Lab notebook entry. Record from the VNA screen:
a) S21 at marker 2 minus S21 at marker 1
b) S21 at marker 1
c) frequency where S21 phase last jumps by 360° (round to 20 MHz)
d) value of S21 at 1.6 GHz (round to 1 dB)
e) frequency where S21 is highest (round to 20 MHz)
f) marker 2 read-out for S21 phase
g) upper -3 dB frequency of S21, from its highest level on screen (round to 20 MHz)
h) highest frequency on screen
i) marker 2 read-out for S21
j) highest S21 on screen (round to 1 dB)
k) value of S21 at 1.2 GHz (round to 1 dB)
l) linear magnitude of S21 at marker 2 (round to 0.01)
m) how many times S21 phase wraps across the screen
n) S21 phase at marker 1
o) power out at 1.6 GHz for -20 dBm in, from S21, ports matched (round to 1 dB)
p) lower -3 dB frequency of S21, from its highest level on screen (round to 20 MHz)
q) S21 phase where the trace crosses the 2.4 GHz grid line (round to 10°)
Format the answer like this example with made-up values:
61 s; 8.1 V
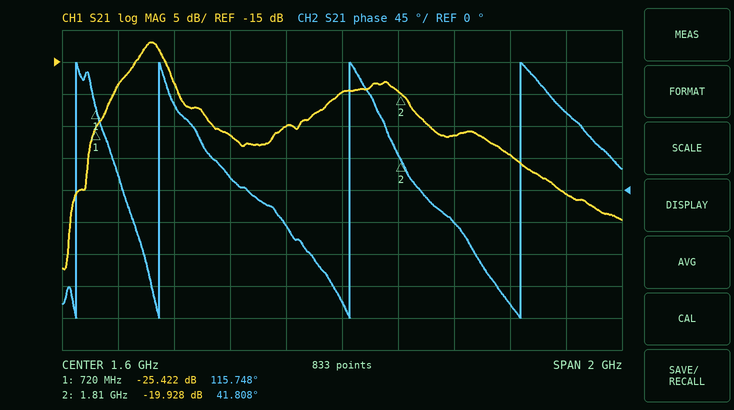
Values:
5.494 dB; -25.422 dB; 2.24 GHz; -20 dB; 920 MHz; 41.808°; 960 MHz; 2.6 GHz; -19.928 dB; -12 dB; -26 dB; 0.10; 4; 115.748°; -40 dBm; 860 MHz; 110°
